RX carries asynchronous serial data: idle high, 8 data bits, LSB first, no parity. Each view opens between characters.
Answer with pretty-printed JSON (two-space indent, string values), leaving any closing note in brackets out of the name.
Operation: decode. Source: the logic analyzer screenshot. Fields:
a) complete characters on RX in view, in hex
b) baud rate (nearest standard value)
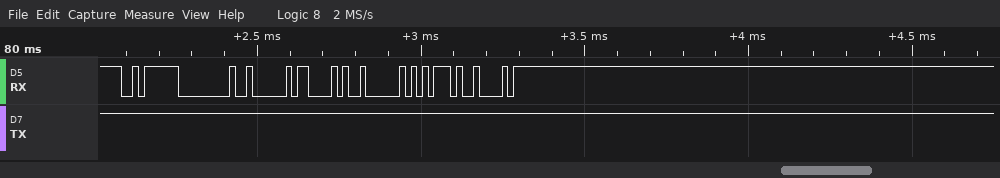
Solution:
{
  "complete characters on RX in view, in hex": "FA, 00, 02, 43, 02, 75, 42",
  "baud rate": "57600 baud"
}
